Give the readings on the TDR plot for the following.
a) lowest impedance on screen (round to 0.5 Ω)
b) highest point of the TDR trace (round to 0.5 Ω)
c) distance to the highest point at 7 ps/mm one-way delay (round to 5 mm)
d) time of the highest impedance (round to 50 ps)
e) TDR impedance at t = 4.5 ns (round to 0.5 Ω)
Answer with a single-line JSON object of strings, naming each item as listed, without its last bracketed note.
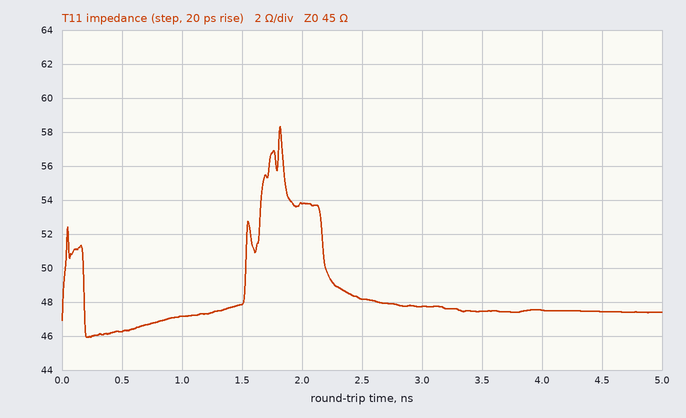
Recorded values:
{"lowest impedance on screen": "46.0 Ω", "highest point of the TDR trace": "58.5 Ω", "distance to the highest point at 7 ps/mm one-way delay": "130 mm", "time of the highest impedance": "1.80 ns", "TDR impedance at t = 4.5 ns": "47.5 Ω"}
